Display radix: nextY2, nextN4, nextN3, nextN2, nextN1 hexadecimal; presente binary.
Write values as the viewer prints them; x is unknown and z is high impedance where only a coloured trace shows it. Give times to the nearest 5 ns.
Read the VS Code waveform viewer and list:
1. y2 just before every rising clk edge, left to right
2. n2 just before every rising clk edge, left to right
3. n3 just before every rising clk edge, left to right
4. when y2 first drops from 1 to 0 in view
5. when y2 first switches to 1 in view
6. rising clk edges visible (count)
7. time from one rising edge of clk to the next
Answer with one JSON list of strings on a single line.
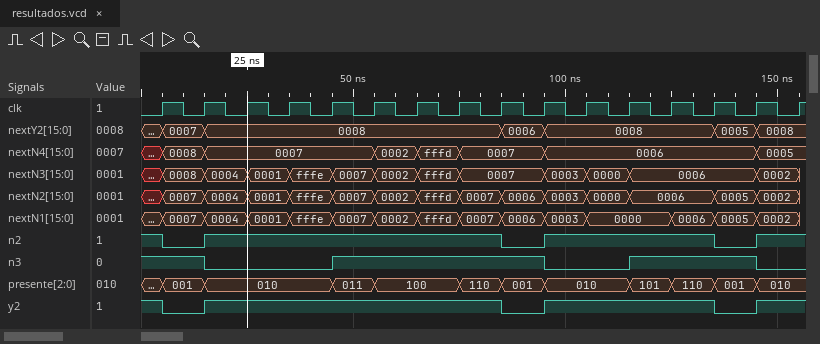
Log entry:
["1 0 1 1 1 1 1 1 1 0 1 1 1 1 0 1", "1 0 1 1 1 1 1 1 1 0 1 1 1 1 0 1", "1 1 0 0 0 1 1 1 1 1 0 0 1 1 1 0", "5 ns", "15 ns", "16", "10 ns"]
